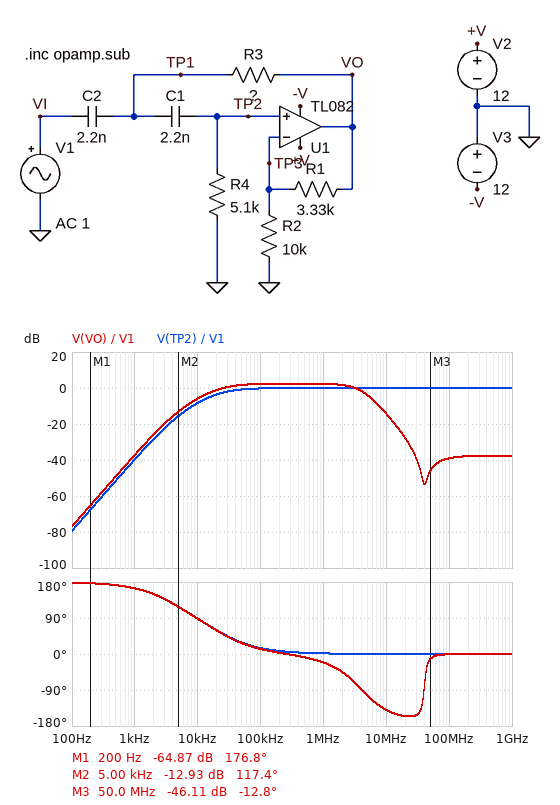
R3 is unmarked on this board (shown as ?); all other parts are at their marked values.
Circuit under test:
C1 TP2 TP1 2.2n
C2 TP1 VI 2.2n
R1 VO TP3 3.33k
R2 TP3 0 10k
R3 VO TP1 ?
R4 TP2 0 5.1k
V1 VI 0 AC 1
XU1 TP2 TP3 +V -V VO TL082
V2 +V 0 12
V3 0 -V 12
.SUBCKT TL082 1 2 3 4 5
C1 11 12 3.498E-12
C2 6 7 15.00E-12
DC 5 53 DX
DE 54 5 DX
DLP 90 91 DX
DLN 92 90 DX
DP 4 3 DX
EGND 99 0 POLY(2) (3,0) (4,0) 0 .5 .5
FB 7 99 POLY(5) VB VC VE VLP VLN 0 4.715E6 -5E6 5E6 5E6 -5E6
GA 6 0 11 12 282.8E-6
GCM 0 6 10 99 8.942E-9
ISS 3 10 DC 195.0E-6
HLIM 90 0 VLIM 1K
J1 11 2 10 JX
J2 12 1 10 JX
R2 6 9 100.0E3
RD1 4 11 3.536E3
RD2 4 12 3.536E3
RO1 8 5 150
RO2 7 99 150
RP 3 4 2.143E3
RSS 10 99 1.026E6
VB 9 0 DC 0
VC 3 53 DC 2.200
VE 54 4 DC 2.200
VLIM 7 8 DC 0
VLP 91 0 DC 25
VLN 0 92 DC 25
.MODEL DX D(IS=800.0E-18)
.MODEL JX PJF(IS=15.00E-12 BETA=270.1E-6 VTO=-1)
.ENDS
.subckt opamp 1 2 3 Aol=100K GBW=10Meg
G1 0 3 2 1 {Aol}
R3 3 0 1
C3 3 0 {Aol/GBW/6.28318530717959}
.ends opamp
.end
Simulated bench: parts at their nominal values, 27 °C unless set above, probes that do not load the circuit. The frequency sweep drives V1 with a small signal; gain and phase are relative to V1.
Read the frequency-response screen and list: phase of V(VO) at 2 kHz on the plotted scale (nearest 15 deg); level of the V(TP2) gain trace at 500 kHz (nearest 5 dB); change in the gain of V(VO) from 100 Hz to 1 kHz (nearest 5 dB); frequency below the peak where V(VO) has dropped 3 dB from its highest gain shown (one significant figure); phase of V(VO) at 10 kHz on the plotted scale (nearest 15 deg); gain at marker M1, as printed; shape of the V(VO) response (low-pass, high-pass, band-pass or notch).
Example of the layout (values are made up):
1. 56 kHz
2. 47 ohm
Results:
1. 150 deg
2. 0 dB
3. 40 dB
4. 20 kHz
5. 90 deg
6. -64.87 dB
7. band-pass
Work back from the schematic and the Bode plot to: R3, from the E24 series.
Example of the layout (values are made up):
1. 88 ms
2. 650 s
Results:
1. 11 kΩ
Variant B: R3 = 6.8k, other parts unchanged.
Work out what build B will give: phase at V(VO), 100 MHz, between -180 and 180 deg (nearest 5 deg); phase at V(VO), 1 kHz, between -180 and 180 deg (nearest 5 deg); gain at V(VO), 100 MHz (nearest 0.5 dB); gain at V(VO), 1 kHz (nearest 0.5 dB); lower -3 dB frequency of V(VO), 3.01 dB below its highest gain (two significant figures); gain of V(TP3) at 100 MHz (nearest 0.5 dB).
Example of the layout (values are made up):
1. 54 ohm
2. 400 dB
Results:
1. 0 deg
2. 170 deg
3. -34.5 dB
4. -41.0 dB
5. 19 kHz
6. -37.0 dB
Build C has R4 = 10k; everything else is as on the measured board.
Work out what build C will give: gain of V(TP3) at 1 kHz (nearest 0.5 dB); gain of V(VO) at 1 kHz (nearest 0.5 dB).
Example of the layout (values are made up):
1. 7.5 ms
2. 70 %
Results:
1. -33.5 dB
2. -31.0 dB
